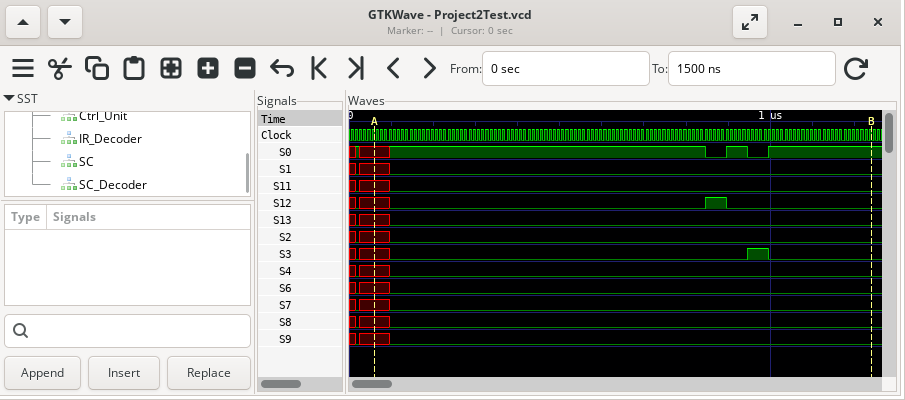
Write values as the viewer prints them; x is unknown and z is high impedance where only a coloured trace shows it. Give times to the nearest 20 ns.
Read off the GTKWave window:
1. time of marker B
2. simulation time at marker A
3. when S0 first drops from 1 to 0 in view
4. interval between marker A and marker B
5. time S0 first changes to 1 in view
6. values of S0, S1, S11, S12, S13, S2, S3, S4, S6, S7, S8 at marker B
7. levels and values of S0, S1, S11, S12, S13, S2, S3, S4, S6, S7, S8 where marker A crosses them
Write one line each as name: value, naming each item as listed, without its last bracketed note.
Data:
time of marker B: 1240 ns
simulation time at marker A: 60 ns
when S0 first drops from 1 to 0 in view: 840 ns
interval between marker A and marker B: 1180 ns
time S0 first changes to 1 in view: 20 ns
values of S0, S1, S11, S12, S13, S2, S3, S4, S6, S7, S8 at marker B: S0=1, S1=0, S11=0, S12=0, S13=0, S2=0, S3=0, S4=0, S6=0, S7=0, S8=0
levels and values of S0, S1, S11, S12, S13, S2, S3, S4, S6, S7, S8 where marker A crosses them: S0=x, S1=x, S11=x, S12=x, S13=x, S2=x, S3=x, S4=x, S6=x, S7=x, S8=x
